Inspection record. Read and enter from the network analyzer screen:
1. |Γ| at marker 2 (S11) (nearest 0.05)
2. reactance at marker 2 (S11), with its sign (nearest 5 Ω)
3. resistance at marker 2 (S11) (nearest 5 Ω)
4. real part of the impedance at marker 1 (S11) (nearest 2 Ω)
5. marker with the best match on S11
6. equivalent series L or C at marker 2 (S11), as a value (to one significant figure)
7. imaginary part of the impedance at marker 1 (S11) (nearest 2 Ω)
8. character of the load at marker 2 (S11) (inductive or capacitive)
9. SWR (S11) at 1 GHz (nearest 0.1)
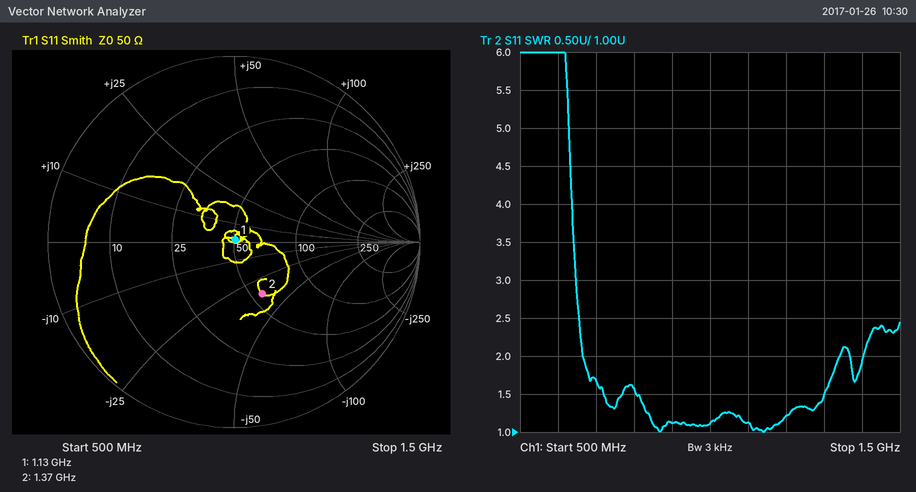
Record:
0.30
-35 Ω
55 Ω
50 Ω
marker 1
3 pF
+2 Ω
capacitive
1.1
